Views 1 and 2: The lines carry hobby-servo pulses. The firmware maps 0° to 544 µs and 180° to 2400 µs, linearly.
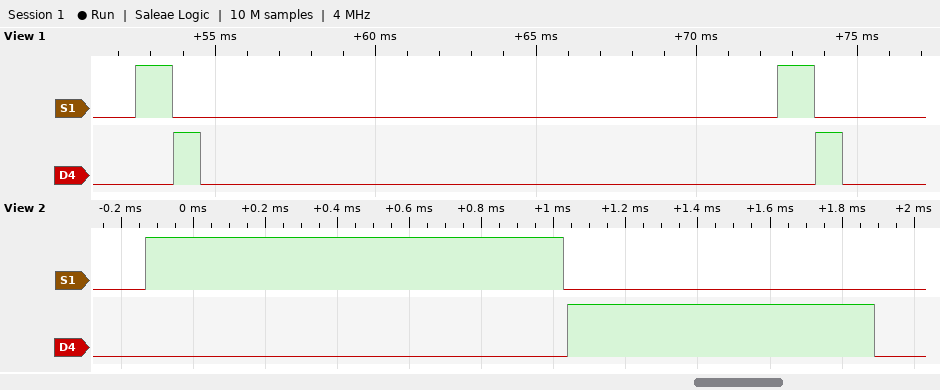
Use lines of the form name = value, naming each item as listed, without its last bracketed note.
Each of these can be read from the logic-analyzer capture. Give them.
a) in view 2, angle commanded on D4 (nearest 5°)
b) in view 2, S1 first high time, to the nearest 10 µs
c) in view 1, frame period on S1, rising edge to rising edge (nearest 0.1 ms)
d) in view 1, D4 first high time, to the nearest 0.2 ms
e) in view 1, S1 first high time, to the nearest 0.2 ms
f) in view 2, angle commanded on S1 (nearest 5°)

in view 2, angle commanded on D4 = 30°
in view 2, S1 first high time, to the nearest 10 µs = 1160 µs
in view 1, frame period on S1, rising edge to rising edge = 20.0 ms
in view 1, D4 first high time, to the nearest 0.2 ms = 0.8 ms
in view 1, S1 first high time, to the nearest 0.2 ms = 1.2 ms
in view 2, angle commanded on S1 = 60°
